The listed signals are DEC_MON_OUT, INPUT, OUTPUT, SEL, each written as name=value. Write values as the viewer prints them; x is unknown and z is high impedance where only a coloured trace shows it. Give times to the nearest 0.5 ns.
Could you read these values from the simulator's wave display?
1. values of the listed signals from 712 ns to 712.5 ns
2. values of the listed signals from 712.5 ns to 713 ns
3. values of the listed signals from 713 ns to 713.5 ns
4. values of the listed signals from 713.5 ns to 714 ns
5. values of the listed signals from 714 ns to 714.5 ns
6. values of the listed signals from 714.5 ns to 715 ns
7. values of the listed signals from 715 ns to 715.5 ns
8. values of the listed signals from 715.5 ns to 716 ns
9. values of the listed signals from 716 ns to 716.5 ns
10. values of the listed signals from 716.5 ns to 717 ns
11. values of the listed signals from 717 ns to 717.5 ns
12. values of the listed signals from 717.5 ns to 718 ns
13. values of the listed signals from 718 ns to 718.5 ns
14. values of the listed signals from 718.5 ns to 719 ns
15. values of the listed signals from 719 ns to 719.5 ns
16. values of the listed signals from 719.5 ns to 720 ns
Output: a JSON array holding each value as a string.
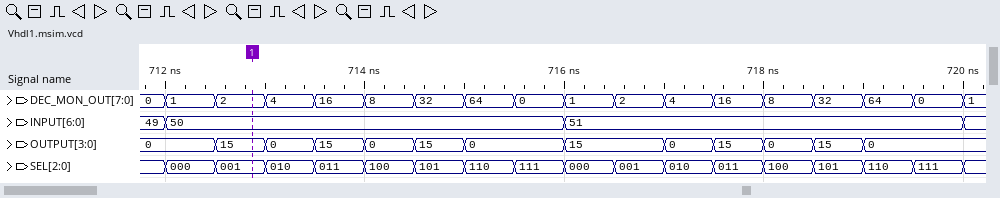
["DEC_MON_OUT=1, INPUT=50, OUTPUT=0, SEL=000", "DEC_MON_OUT=2, INPUT=50, OUTPUT=15, SEL=001", "DEC_MON_OUT=4, INPUT=50, OUTPUT=0, SEL=010", "DEC_MON_OUT=16, INPUT=50, OUTPUT=15, SEL=011", "DEC_MON_OUT=8, INPUT=50, OUTPUT=0, SEL=100", "DEC_MON_OUT=32, INPUT=50, OUTPUT=15, SEL=101", "DEC_MON_OUT=64, INPUT=50, OUTPUT=0, SEL=110", "DEC_MON_OUT=0, INPUT=50, OUTPUT=0, SEL=111", "DEC_MON_OUT=1, INPUT=51, OUTPUT=15, SEL=000", "DEC_MON_OUT=2, INPUT=51, OUTPUT=15, SEL=001", "DEC_MON_OUT=4, INPUT=51, OUTPUT=0, SEL=010", "DEC_MON_OUT=16, INPUT=51, OUTPUT=15, SEL=011", "DEC_MON_OUT=8, INPUT=51, OUTPUT=0, SEL=100", "DEC_MON_OUT=32, INPUT=51, OUTPUT=15, SEL=101", "DEC_MON_OUT=64, INPUT=51, OUTPUT=0, SEL=110", "DEC_MON_OUT=0, INPUT=51, OUTPUT=0, SEL=111"]
